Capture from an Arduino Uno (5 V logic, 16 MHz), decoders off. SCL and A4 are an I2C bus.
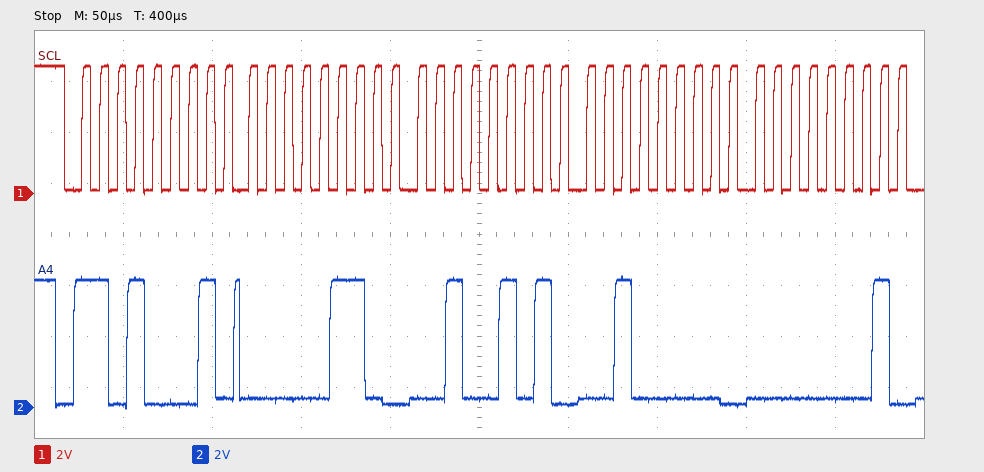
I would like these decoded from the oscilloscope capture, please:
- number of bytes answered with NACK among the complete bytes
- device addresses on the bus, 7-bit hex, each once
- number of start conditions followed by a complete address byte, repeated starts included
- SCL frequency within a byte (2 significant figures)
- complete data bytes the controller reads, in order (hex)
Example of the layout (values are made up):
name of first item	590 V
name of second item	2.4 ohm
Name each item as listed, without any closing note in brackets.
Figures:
number of bytes answered with NACK among the complete bytes	0
device addresses on the bus, 7-bit hex, each once	0x68
number of start conditions followed by a complete address byte, repeated starts included	1
SCL frequency within a byte	100 kHz
complete data bytes the controller reads, in order	06 25 20 01
